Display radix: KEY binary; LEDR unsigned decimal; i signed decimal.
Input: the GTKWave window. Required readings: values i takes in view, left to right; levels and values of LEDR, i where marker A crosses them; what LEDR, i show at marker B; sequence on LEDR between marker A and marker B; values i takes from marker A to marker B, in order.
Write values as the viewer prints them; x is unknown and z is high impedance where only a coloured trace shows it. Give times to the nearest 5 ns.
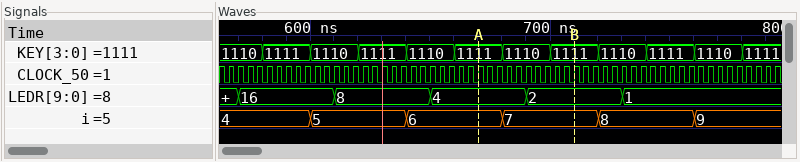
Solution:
4, 5, 6, 7, 8, 9
LEDR=4, i=6
LEDR=2, i=7
4, 2
6, 7
